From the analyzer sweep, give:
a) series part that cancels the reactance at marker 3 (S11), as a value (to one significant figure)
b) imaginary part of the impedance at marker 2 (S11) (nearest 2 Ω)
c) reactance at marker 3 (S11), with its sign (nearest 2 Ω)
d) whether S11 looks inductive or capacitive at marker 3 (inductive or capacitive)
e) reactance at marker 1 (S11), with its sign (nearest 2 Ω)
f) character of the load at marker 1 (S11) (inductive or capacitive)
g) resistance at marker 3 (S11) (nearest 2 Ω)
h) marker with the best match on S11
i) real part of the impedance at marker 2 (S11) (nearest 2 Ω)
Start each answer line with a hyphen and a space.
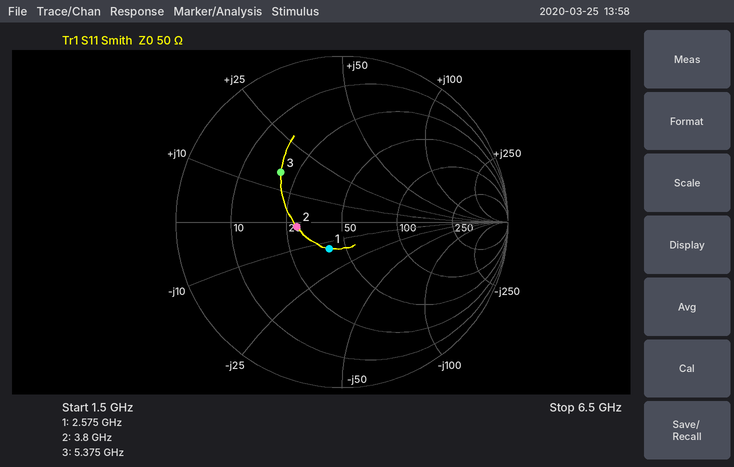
- 2 pF
- -2 Ω
- +16 Ω
- inductive
- -14 Ω
- capacitive
- 20 Ω
- marker 1
- 28 Ω
